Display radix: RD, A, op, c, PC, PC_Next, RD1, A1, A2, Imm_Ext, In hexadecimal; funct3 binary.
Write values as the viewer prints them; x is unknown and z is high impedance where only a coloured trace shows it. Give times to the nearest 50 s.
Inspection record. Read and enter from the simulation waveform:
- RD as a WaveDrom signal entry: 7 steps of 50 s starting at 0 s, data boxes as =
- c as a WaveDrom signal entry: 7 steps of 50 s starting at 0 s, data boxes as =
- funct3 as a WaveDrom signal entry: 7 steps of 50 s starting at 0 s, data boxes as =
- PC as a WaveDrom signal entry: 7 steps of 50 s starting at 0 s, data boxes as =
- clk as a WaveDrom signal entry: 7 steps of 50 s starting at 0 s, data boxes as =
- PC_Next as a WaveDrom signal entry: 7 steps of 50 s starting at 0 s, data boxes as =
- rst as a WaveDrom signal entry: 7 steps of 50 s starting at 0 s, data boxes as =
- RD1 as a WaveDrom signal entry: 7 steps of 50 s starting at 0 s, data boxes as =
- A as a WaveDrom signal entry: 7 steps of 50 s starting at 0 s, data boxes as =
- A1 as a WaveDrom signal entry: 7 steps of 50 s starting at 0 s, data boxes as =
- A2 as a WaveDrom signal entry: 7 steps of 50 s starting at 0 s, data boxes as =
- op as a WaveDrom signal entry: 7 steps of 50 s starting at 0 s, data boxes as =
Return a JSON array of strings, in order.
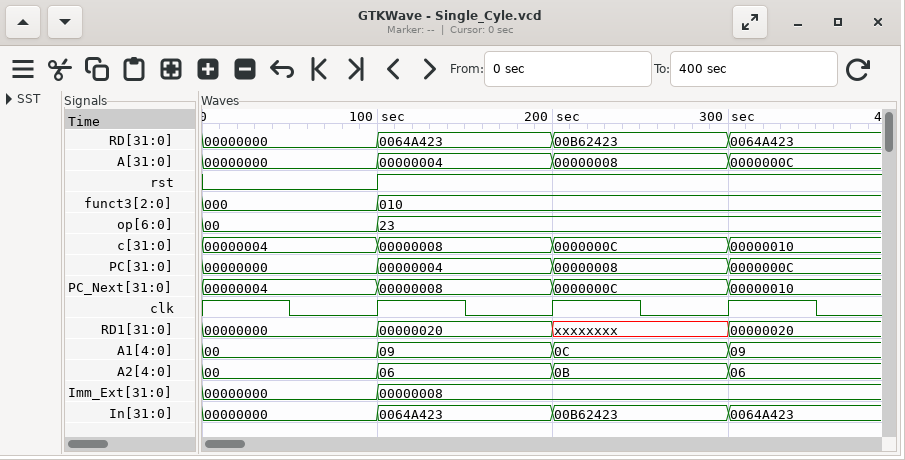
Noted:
["{name: 'RD', wave: '=.=.=.=', data: '00000000 0064A423 00B62423 0064A423'}", "{name: 'c', wave: '=.=.=.=', data: '00000004 00000008 0000000C 00000010'}", "{name: 'funct3', wave: '=.=....', data: '000 010'}", "{name: 'PC', wave: '=.=.=.=', data: '00000000 00000004 00000008 0000000C'}", "{name: 'clk', wave: '1010101'}", "{name: 'PC_Next', wave: '=.=.=.=', data: '00000004 00000008 0000000C 00000010'}", "{name: 'rst', wave: '0.1....'}", "{name: 'RD1', wave: '=.=.x.=', data: '00000000 00000020 00000020'}", "{name: 'A', wave: '=.=.=.=', data: '00000000 00000004 00000008 0000000C'}", "{name: 'A1', wave: '=.=.=.=', data: '00 09 0C 09'}", "{name: 'A2', wave: '=.=.=.=', data: '00 06 0B 06'}", "{name: 'op', wave: '=.=....', data: '00 23'}"]
